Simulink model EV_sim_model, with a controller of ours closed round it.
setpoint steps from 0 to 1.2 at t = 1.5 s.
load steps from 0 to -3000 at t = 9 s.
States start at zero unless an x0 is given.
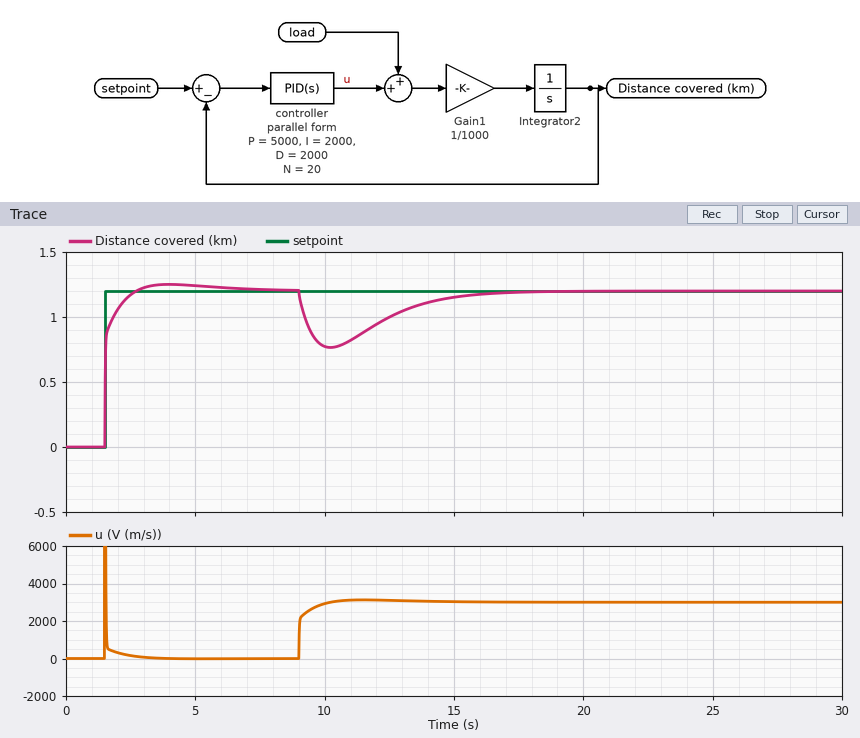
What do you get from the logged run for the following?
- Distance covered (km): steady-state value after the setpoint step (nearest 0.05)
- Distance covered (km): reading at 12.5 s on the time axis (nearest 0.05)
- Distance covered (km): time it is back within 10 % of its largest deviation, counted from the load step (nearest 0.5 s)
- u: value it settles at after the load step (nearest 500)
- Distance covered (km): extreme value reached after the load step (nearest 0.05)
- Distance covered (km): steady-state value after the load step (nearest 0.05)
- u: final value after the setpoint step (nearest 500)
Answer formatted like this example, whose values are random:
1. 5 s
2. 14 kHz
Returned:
1. 1.20
2. 1.00
3. 6.0 s
4. 3000
5. 0.75
6. 1.20
7. 0
